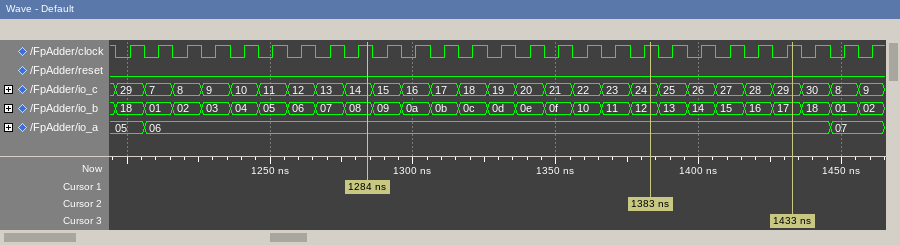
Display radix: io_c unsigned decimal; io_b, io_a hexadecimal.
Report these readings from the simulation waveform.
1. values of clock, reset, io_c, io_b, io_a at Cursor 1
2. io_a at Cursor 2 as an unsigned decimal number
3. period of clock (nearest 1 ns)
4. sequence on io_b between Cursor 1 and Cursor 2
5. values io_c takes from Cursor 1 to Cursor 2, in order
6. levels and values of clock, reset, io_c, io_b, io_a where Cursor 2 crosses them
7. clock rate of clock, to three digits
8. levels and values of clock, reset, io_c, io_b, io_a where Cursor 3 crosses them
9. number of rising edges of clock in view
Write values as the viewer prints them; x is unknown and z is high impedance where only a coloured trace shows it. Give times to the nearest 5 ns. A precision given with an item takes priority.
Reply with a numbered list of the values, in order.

1. clock=1, reset=0, io_c=14, io_b=08, io_a=06
2. 6
3. 10 ns
4. 08, 09, 0a, 0b, 0c, 0d, 0e, 0f, 10, 11, 12
5. 14, 15, 16, 17, 18, 19, 20, 21, 22, 23, 24
6. clock=1, reset=0, io_c=24, io_b=12, io_a=06
7. 100 MHz
8. clock=1, reset=0, io_c=29, io_b=17, io_a=06
9. 27
